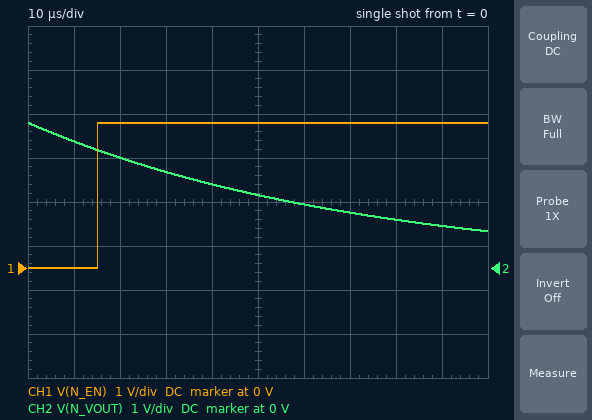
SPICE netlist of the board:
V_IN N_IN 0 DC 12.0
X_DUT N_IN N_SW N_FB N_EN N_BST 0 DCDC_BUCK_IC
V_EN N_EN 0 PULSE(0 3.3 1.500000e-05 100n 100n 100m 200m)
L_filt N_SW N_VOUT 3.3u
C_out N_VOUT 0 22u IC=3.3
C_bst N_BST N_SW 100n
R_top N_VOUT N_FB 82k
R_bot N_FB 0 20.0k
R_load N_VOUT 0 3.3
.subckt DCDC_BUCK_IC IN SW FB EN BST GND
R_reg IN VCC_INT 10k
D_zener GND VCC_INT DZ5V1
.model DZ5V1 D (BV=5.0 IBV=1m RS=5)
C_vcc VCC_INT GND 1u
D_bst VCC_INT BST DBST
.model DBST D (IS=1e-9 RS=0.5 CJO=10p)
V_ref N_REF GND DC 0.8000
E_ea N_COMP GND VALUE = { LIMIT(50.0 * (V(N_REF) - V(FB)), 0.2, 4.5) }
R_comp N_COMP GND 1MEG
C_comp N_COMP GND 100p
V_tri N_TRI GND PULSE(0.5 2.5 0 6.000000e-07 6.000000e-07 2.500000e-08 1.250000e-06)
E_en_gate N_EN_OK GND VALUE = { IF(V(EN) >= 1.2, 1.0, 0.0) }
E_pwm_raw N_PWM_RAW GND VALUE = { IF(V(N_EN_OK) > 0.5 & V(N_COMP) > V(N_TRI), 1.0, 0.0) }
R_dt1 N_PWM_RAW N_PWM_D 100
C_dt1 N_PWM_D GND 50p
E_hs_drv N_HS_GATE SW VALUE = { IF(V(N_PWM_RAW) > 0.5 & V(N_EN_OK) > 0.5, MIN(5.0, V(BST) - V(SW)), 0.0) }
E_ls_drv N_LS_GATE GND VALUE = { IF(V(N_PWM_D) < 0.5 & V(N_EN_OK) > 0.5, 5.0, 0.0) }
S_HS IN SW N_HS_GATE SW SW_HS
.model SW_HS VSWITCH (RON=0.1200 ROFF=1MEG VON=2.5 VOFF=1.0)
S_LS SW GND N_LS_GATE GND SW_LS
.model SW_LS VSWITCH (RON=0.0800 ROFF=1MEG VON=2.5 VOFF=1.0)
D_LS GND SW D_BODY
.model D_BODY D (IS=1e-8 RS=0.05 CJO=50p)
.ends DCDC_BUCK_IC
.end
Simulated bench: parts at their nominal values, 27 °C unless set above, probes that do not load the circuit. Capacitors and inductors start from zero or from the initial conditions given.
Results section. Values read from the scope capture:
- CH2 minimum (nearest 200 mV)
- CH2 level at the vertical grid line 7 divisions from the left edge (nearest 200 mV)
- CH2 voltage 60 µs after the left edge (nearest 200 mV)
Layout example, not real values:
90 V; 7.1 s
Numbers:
800 mV; 1.2 V; 1.4 V
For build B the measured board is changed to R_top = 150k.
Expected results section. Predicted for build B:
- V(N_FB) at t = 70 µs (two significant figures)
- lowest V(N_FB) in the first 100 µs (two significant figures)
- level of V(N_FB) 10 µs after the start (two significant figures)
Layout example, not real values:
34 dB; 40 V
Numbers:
150 mV; 98 mV; 340 mV
